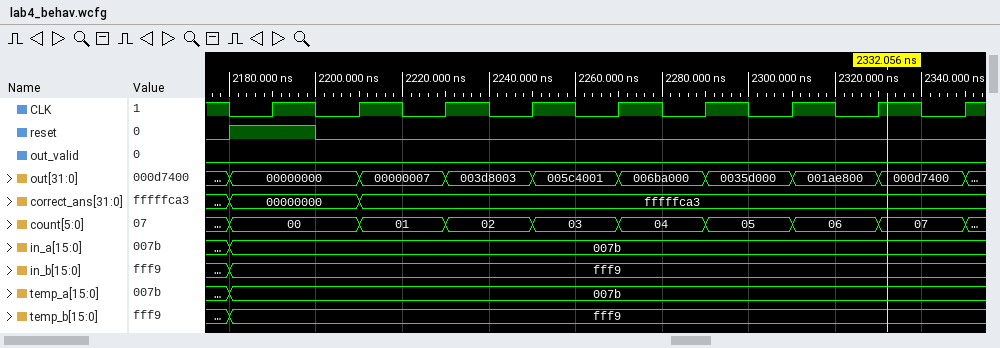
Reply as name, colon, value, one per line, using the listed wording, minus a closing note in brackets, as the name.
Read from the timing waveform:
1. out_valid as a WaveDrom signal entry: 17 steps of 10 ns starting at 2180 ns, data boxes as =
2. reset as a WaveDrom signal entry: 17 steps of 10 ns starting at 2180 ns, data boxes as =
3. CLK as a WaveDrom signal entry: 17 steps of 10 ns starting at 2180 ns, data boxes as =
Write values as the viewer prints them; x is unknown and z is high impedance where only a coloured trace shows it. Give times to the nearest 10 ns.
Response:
out_valid as a WaveDrom signal entry: 17 steps of 10 ns starting at 2180 ns, data boxes as =: {name: 'out_valid', wave: '0................'}
reset as a WaveDrom signal entry: 17 steps of 10 ns starting at 2180 ns, data boxes as =: {name: 'reset', wave: '1.0..............'}
CLK as a WaveDrom signal entry: 17 steps of 10 ns starting at 2180 ns, data boxes as =: {name: 'CLK', wave: '01010101010101010'}
